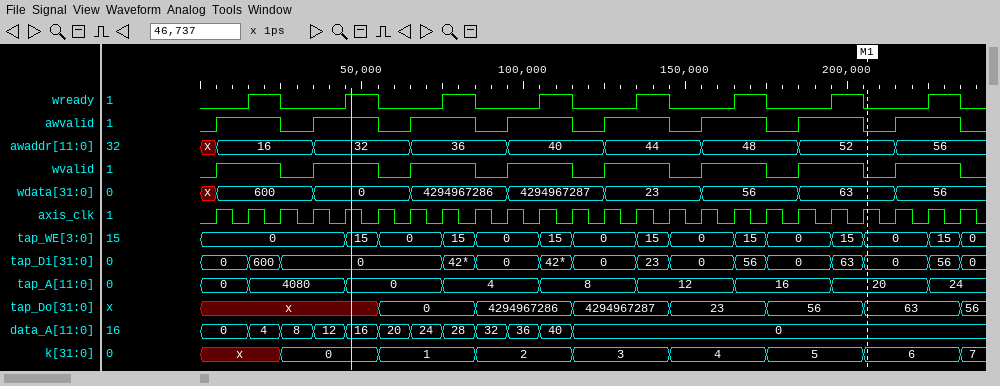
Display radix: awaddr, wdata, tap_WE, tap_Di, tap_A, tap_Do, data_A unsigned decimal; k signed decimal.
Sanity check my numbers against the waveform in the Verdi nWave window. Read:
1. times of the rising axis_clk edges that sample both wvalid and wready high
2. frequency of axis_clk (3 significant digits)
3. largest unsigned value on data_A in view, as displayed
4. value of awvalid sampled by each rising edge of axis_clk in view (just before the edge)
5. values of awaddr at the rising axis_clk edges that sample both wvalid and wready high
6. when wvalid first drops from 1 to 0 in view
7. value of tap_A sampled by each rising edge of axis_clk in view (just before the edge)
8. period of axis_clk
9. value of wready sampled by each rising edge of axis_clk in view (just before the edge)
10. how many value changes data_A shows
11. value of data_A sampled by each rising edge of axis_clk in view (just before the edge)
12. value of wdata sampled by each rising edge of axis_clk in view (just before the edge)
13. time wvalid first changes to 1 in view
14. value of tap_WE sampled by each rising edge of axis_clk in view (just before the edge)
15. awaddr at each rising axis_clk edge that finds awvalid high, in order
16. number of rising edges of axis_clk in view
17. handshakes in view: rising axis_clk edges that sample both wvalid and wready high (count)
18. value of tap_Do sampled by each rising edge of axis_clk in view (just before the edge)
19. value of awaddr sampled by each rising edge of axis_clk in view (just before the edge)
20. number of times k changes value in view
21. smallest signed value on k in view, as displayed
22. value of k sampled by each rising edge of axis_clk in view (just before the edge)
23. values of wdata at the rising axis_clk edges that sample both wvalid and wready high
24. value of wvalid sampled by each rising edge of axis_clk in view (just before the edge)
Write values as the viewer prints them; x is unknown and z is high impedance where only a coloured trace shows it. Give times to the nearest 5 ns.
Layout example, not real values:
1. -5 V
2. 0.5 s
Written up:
1. 25 ns, 55 ns, 85 ns, 115 ns, 145 ns, 175 ns, 205 ns, 235 ns
2. 100 MHz
3. 40
4. 0 1 1 0 1 1 0 1 1 0 1 1 0 1 1 0 1 1 0 1 1 0 1 1
5. 16, 32, 36, 40, 44, 48, 52, 56
6. 25 ns
7. 0, 0, 4080, 4080, 4080, 0, 0, 0, 4, 4, 4, 8, 8, 8, 12, 12, 12, 16, 16, 16, 20, 20, 20, 24
8. 10 ns
9. 0 0 1 0 0 1 0 0 1 0 0 1 0 0 1 0 0 1 0 0 1 0 0 1
10. 11
11. 0, 0, 4, 8, 12, 16, 20, 24, 28, 32, 36, 40, 0, 0, 0, 0, 0, 0, 0, 0, 0, 0, 0, 0
12. x, 600, 600, 600, 0, 0, 0, 4294967286, 4294967286, 4294967286, 4294967287, 4294967287, 4294967287, 23, 23, 23, 56, 56, 56, 63, 63, 63, 56, 56
13. 5 ns
14. 0, 0, 0, 0, 0, 15, 0, 0, 15, 0, 0, 15, 0, 0, 15, 0, 0, 15, 0, 0, 15, 0, 0, 15
15. 16, 16, 32, 32, 36, 36, 40, 40, 44, 44, 48, 48, 52, 52, 56, 56
16. 24
17. 8
18. x, x, x, x, x, x, 0, 0, 0, 4294967286, 4294967286, 4294967286, 4294967287, 4294967287, 4294967287, 23, 23, 23, 56, 56, 56, 63, 63, 63
19. x, 16, 16, 16, 32, 32, 32, 36, 36, 36, 40, 40, 40, 44, 44, 44, 48, 48, 48, 52, 52, 52, 56, 56
20. 8
21. 0
22. x, x, x, 0, 0, 0, 1, 1, 1, 2, 2, 2, 3, 3, 3, 4, 4, 4, 5, 5, 5, 6, 6, 6
23. 600, 0, 4294967286, 4294967287, 23, 56, 63, 56
24. 0 1 1 0 1 1 0 1 1 0 1 1 0 1 1 0 1 1 0 1 1 0 1 1
